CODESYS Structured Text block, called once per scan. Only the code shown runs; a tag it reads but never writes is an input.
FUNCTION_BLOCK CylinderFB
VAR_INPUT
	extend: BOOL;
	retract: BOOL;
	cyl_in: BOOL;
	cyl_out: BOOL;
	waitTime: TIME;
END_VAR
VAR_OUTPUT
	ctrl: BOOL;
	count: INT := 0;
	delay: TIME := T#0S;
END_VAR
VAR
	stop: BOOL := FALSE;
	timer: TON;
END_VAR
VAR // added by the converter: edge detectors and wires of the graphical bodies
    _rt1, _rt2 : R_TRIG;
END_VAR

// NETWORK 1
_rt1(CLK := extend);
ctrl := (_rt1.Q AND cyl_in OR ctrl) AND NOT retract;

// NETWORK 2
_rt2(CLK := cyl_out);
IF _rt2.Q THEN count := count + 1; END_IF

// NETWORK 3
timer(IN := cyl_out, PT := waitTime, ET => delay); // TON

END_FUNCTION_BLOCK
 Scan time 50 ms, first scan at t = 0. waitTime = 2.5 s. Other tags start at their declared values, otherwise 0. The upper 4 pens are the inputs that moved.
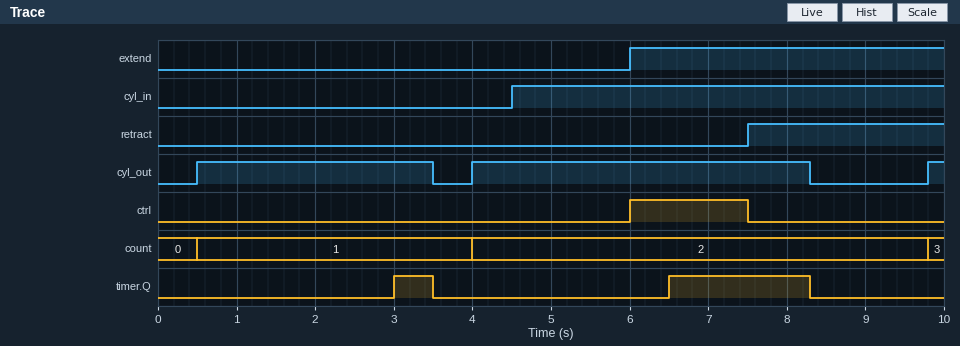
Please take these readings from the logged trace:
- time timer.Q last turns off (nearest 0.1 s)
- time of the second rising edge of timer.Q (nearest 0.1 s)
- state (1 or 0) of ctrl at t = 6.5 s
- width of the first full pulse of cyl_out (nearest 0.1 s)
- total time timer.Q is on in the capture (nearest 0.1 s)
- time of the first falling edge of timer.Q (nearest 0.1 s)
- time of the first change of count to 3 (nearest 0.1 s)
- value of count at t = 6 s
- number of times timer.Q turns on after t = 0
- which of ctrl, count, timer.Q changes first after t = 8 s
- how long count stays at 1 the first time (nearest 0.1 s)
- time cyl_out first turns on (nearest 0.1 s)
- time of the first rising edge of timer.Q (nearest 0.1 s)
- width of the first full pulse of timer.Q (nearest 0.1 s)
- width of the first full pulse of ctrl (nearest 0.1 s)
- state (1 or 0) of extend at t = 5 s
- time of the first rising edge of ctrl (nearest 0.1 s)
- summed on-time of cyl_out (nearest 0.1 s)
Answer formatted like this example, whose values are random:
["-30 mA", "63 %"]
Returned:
["8.3 s", "6.5 s", "1", "3.0 s", "2.3 s", "3.5 s", "9.8 s", "2", "2", "timer.Q", "3.5 s", "0.5 s", "3.0 s", "0.5 s", "1.5 s", "0", "6.0 s", "7.5 s"]
